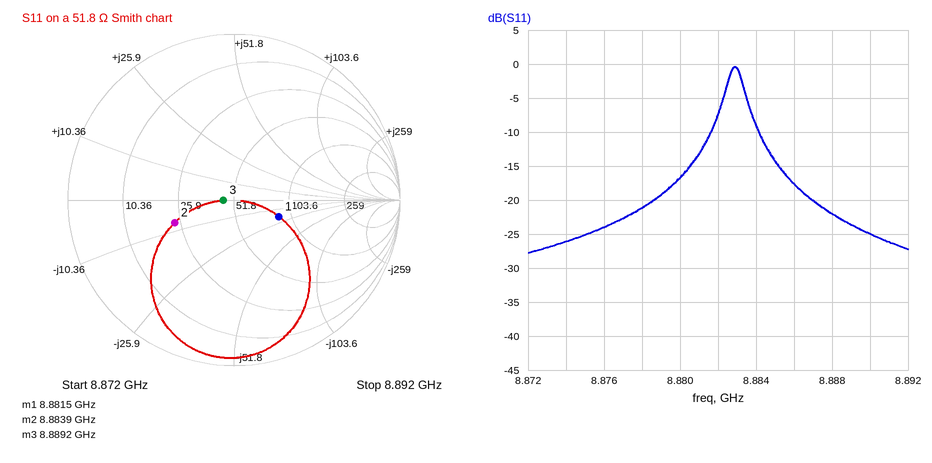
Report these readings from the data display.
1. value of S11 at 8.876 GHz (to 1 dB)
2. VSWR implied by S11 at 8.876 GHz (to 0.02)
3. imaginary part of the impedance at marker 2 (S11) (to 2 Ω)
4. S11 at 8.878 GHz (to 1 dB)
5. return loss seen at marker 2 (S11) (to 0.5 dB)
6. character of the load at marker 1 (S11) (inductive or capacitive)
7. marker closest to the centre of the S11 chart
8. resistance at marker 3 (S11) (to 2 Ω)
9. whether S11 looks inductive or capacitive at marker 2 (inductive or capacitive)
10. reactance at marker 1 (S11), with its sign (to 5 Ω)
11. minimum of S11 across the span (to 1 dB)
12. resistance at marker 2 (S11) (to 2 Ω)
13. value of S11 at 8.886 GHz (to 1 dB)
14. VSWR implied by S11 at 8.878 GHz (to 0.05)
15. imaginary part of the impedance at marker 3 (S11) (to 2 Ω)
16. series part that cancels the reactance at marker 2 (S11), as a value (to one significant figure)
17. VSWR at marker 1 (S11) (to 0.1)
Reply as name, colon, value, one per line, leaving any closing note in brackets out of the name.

value of S11 at 8.876 GHz: -24 dB
VSWR implied by S11 at 8.876 GHz: 1.14
imaginary part of the impedance at marker 2 (S11): -8 Ω
S11 at 8.878 GHz: -21 dB
return loss seen at marker 2 (S11): 8.5 dB
character of the load at marker 1 (S11): capacitive
marker closest to the centre of the S11 chart: marker 3
resistance at marker 3 (S11): 46 Ω
whether S11 looks inductive or capacitive at marker 2: capacitive
reactance at marker 1 (S11), with its sign: -20 Ω
minimum of S11 across the span: -28 dB
resistance at marker 2 (S11): 24 Ω
value of S11 at 8.886 GHz: -18 dB
VSWR implied by S11 at 8.878 GHz: 1.20
imaginary part of the impedance at marker 3 (S11): 0 Ω
series part that cancels the reactance at marker 2 (S11), as a value: 100 pH
VSWR at marker 1 (S11): 1.8
